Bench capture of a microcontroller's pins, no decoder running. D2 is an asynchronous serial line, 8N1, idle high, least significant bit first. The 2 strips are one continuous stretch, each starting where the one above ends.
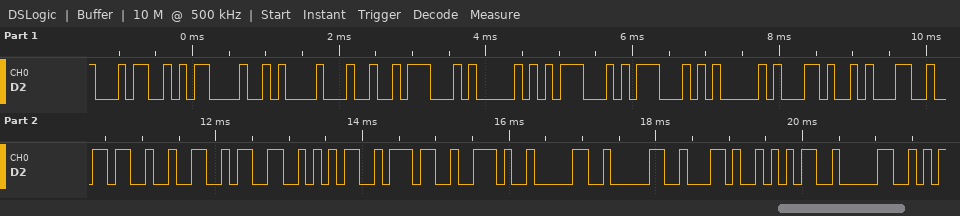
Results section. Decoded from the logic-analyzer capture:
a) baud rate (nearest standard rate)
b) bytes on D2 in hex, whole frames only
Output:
9600 baud
0x34 0x0D 0x0A 0x24 0x47 0x50 0x47 0x47 0x41 0x2C 0x31 0x36 0x32 0x33 0x35 0x37 0x2E 0x30 0x30 0x2C 0x35 0x30
